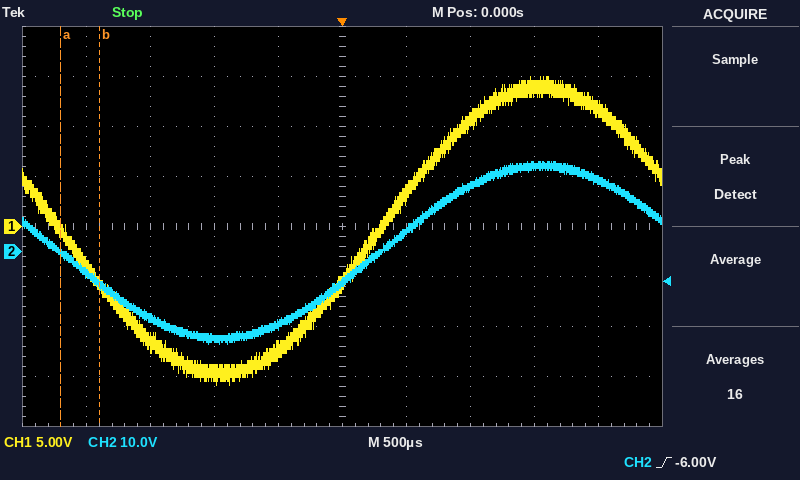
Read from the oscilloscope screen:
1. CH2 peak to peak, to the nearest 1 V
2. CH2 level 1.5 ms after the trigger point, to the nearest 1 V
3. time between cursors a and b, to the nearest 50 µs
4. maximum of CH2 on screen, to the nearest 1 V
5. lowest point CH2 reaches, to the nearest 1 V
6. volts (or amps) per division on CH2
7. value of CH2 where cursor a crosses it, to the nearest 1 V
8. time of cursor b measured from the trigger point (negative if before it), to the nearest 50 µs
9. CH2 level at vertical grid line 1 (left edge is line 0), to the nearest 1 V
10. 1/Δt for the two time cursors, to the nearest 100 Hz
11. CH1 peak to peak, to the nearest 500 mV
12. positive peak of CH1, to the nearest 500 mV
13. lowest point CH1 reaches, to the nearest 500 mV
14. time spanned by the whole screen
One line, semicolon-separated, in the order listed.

36 V; 17 V; 300 µs; 18 V; -18 V; 10 V; 0 V; -1.90 ms; -4 V; 3.3 kHz; 31.0 V; 15.0 V; -16.0 V; 5 ms
